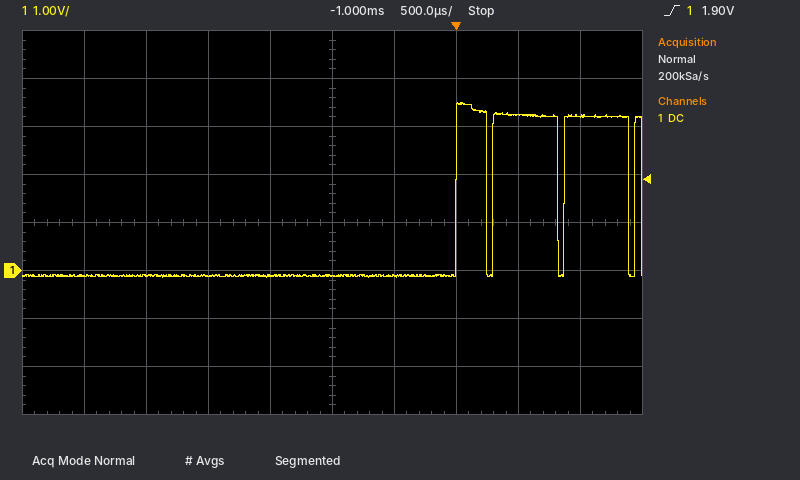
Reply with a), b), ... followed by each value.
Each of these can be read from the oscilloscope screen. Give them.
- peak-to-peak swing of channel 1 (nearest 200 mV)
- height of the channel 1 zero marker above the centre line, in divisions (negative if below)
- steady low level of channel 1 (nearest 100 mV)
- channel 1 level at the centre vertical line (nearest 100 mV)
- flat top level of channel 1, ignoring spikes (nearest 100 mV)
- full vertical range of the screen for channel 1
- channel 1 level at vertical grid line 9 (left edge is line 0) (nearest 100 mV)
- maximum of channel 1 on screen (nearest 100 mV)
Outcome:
a) 3.6 V
b) -1.0 div
c) -100 mV
d) -100 mV
e) 3.2 V
f) 8 V
g) 3.2 V
h) 3.5 V
